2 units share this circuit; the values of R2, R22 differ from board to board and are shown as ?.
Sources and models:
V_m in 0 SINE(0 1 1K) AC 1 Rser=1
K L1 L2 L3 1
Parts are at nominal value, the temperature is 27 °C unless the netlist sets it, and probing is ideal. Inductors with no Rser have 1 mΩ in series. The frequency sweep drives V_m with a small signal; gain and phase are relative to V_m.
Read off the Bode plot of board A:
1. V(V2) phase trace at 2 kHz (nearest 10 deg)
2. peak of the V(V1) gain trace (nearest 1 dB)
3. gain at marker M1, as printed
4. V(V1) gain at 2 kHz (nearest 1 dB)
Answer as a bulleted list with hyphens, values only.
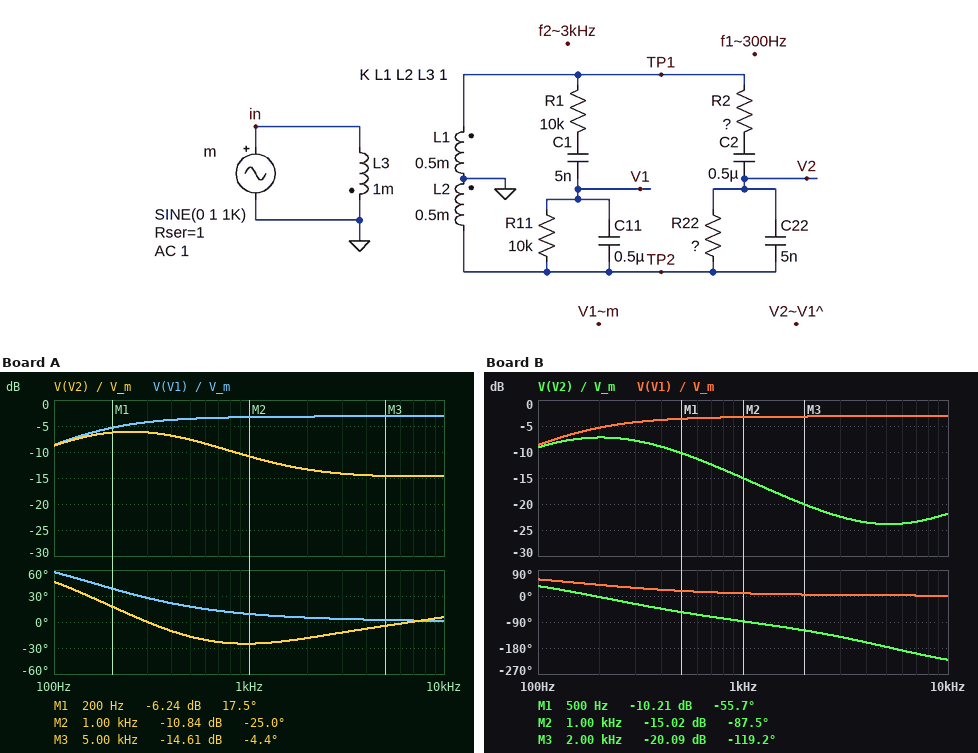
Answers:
- -20 deg
- -3 dB
- -6.24 dB
- -3 dB
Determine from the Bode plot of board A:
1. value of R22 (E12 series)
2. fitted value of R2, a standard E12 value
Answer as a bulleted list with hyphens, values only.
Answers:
- 330 Ω
- 560 Ω
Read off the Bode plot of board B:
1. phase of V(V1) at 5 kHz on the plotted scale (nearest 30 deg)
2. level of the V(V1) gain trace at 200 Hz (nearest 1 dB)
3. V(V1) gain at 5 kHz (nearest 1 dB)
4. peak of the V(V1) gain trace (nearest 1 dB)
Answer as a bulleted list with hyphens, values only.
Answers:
- 0 deg
- -5 dB
- -3 dB
- -3 dB
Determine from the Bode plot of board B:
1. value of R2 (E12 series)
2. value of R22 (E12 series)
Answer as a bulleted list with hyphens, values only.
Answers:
- 560 Ω
- 680 Ω
